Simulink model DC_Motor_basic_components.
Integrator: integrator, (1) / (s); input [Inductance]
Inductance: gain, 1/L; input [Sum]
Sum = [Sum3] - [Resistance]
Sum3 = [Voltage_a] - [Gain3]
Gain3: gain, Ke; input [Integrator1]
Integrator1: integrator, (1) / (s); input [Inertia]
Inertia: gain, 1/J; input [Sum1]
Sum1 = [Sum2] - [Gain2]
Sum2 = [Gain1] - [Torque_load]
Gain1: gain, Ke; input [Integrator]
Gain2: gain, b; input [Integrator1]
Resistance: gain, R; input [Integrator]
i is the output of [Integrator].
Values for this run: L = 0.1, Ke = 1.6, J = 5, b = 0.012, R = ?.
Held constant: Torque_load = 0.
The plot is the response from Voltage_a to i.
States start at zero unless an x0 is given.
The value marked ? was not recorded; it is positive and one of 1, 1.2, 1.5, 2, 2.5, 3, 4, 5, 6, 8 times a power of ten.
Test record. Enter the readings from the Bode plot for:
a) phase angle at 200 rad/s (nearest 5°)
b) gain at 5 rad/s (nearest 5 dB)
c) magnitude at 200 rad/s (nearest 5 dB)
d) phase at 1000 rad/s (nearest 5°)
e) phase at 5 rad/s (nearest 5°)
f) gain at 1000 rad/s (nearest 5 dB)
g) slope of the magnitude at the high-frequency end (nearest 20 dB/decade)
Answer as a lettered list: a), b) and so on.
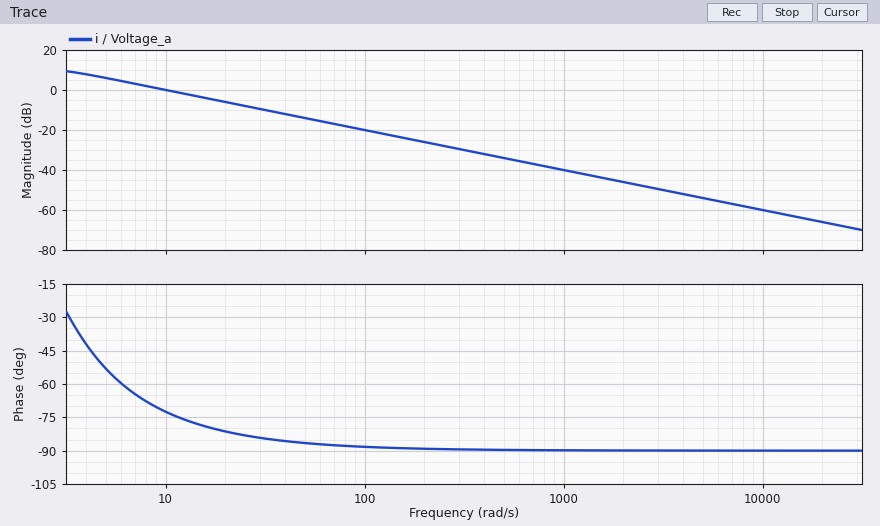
a) -90°
b) 5 dB
c) -25 dB
d) -90°
e) -55°
f) -40 dB
g) -20 dB/decade
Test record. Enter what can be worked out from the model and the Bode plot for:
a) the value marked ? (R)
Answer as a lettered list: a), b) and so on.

a) 0.3
